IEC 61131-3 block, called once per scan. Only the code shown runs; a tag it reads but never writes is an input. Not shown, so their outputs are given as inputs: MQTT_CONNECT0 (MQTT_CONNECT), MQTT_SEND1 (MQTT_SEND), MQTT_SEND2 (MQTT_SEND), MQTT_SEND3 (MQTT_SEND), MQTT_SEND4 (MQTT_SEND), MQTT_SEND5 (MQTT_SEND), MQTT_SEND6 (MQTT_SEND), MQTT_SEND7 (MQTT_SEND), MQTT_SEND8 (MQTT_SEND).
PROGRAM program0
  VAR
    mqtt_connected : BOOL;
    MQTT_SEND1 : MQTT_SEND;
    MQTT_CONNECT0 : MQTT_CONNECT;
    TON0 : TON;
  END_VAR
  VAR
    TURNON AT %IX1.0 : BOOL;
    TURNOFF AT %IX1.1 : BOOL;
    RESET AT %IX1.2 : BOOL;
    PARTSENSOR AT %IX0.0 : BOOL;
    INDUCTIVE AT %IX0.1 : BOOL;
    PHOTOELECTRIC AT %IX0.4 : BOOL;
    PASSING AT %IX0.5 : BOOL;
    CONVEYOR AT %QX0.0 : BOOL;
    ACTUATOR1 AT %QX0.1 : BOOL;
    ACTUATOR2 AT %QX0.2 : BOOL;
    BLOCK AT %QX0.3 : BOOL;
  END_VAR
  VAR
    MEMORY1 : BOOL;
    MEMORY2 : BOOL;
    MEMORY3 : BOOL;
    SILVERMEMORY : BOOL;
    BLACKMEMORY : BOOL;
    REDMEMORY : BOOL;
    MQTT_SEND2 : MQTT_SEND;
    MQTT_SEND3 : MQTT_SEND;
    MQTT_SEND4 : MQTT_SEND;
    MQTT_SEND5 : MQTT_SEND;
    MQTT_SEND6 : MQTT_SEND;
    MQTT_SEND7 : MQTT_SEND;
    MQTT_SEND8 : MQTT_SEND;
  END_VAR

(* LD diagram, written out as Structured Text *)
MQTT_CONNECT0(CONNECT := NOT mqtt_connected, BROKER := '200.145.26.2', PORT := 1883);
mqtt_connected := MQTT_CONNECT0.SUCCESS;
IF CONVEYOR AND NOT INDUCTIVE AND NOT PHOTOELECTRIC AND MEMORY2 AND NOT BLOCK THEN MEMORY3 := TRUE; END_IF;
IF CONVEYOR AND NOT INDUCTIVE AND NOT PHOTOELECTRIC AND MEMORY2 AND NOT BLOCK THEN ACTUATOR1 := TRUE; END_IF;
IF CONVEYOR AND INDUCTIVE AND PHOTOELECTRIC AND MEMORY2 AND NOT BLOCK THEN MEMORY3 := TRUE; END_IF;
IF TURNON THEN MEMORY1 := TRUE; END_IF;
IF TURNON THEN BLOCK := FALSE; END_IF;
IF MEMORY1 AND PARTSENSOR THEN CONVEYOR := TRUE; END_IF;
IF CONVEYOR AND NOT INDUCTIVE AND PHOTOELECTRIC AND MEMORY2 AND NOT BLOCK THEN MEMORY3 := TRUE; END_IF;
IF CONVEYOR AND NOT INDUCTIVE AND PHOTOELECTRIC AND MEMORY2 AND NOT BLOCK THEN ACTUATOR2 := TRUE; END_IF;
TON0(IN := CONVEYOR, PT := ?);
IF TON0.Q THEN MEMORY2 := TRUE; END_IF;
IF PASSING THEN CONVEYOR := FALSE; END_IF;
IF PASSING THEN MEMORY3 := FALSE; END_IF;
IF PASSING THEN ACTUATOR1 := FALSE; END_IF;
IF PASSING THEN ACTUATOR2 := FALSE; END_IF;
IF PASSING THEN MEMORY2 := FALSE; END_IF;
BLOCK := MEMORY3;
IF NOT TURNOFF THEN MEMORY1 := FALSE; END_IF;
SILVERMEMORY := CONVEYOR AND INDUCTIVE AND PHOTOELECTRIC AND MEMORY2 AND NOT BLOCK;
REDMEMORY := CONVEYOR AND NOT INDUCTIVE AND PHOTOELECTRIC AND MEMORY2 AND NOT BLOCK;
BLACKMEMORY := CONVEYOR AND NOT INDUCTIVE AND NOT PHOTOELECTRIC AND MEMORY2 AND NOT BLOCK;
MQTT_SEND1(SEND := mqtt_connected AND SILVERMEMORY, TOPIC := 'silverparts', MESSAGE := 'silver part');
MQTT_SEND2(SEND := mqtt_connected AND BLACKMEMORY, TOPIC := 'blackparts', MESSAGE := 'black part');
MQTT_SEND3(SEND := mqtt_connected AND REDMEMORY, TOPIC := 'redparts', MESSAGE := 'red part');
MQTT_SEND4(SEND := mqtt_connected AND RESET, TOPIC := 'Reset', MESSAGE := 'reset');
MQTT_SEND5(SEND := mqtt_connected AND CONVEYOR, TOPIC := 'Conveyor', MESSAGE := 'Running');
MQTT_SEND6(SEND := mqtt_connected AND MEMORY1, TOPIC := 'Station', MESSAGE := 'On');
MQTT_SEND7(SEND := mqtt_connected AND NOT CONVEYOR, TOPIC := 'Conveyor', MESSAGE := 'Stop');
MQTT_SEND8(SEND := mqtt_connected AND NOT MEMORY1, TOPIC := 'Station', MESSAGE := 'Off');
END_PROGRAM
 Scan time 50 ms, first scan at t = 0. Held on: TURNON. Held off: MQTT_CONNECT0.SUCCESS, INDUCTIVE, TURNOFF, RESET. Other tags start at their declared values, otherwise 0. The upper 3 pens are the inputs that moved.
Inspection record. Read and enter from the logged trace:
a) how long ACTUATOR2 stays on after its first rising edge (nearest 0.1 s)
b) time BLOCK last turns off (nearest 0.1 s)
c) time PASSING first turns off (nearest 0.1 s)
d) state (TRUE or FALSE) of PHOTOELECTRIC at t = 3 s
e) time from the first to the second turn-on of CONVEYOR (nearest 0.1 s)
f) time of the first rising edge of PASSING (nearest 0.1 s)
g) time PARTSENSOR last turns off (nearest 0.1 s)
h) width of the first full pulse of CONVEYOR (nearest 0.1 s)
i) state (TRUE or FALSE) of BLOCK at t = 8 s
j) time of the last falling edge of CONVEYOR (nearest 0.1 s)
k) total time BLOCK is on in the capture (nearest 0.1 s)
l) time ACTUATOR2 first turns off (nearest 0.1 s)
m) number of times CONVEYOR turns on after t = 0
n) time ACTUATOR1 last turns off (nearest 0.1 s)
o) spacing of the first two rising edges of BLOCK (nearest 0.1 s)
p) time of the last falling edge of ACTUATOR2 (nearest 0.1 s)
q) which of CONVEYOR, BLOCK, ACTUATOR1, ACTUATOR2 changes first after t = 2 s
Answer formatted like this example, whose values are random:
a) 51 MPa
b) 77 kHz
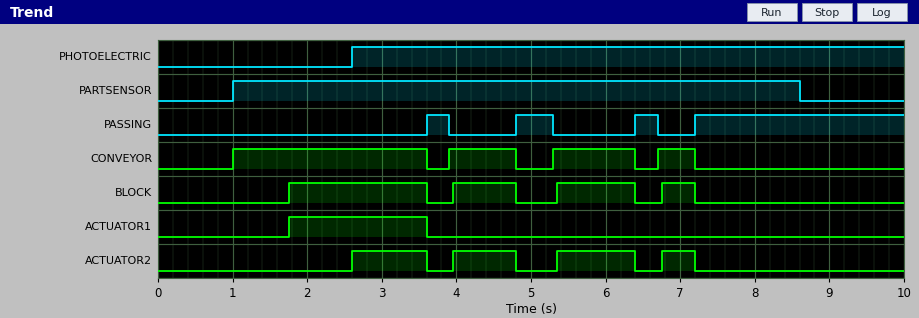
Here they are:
a) 1.0 s
b) 7.2 s
c) 3.9 s
d) TRUE
e) 2.9 s
f) 3.6 s
g) 8.6 s
h) 2.6 s
i) FALSE
j) 7.2 s
k) 4.2 s
l) 3.6 s
m) 4
n) 3.6 s
o) 2.2 s
p) 7.2 s
q) ACTUATOR2
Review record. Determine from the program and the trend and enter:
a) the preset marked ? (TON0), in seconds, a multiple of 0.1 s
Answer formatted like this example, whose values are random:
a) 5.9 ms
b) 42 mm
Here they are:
a) 0.7 s
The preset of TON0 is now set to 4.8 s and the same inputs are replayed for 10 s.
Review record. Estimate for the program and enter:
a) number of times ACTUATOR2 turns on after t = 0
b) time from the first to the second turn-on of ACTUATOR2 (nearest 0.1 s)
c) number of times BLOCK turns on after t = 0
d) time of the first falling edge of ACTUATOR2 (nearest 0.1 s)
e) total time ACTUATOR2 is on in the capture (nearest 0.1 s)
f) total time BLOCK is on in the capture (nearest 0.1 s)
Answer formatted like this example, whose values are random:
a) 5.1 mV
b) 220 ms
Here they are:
a) 2
b) 0.9 s
c) 2
d) 6.4 s
e) 1.0 s
f) 1.0 s
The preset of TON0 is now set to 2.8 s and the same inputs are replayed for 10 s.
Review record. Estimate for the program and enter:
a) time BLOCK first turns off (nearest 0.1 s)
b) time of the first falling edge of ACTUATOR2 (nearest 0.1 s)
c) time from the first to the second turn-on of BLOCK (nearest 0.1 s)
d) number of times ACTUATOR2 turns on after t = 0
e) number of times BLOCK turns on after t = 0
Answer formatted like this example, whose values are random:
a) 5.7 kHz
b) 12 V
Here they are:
a) 4.8 s
b) 4.8 s
c) 1.4 s
d) 3
e) 3
